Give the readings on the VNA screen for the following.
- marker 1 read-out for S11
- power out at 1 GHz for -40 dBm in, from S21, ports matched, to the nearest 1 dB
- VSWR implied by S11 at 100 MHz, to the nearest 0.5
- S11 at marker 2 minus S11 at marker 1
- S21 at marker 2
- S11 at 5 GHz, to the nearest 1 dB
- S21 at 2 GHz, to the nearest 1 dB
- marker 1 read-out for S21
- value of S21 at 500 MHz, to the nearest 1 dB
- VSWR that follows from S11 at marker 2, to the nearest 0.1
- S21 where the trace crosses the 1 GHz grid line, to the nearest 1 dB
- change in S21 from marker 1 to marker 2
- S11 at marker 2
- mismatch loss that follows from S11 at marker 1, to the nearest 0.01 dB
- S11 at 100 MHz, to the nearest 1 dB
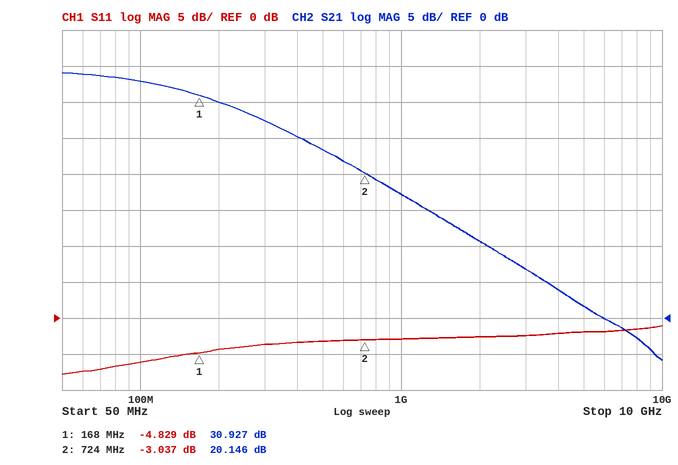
-4.829 dB
-23 dBm
3.0
1.792 dB
20.146 dB
-2 dB
11 dB
30.927 dB
23 dB
5.8
17 dB
-10.781 dB
-3.037 dB
1.73 dB
-6 dB
